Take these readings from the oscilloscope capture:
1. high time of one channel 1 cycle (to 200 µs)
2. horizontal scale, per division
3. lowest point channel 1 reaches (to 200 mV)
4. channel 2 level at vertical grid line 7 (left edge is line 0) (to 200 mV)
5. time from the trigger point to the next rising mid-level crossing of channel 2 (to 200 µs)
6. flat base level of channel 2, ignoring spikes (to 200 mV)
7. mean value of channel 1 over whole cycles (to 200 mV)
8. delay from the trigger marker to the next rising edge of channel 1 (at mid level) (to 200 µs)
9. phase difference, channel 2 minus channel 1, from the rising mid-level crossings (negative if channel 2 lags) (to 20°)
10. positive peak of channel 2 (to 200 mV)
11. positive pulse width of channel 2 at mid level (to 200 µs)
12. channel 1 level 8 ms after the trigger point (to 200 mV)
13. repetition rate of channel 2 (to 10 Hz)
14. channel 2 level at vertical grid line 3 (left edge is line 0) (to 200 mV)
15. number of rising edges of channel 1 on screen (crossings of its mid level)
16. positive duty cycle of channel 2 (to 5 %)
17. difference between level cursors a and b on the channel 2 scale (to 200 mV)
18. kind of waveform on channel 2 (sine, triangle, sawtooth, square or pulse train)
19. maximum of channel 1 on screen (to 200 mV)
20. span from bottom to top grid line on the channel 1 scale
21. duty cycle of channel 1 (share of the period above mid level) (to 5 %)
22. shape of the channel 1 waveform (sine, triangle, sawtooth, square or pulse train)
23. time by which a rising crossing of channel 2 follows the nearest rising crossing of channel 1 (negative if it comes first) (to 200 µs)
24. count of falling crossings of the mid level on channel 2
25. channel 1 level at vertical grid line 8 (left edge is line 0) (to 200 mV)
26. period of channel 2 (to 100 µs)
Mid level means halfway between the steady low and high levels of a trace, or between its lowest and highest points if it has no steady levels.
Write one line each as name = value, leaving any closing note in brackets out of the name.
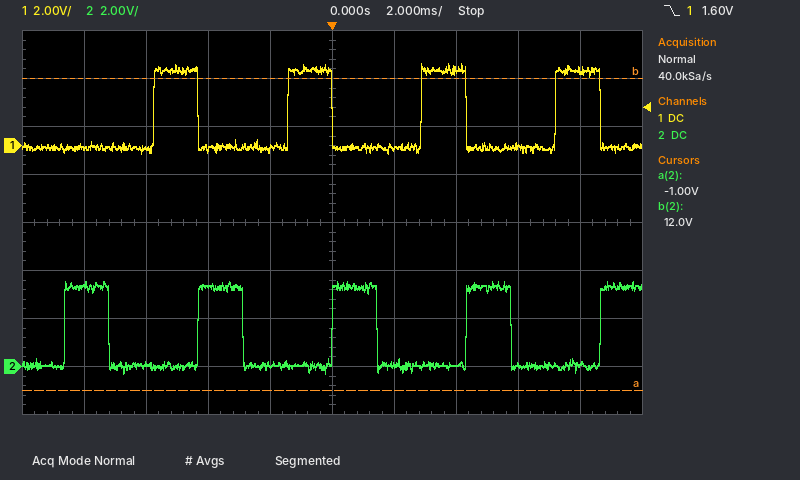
high time of one channel 1 cycle = 1.4 ms
horizontal scale, per division = 2 ms
lowest point channel 1 reaches = -400 mV
channel 2 level at vertical grid line 7 (left edge is line 0) = 0.0 V
time from the trigger point to the next rising mid-level crossing of channel 2 = 4.4 ms
flat base level of channel 2, ignoring spikes = 0.0 V
mean value of channel 1 over whole cycles = 1.0 V
delay from the trigger marker to the next rising edge of channel 1 (at mid level) = 2.8 ms
phase difference, channel 2 minus channel 1, from the rising mid-level crossings (negative if channel 2 lags) = -120°
positive peak of channel 2 = 3.6 V
positive pulse width of channel 2 at mid level = 1.4 ms
channel 1 level 8 ms after the trigger point = 3.2 V
repetition rate of channel 2 = 230 Hz
channel 2 level at vertical grid line 3 (left edge is line 0) = 3.4 V
number of rising edges of channel 1 on screen = 4
positive duty cycle of channel 2 = 35 %
difference between level cursors a and b on the channel 2 scale = 13.0 V
kind of waveform on channel 2 = pulse train
maximum of channel 1 on screen = 3.4 V
span from bottom to top grid line on the channel 1 scale = 16 V
duty cycle of channel 1 (share of the period above mid level) = 35 %
shape of the channel 1 waveform = pulse train
time by which a rising crossing of channel 2 follows the nearest rising crossing of channel 1 (negative if it comes first) = +1.4 ms
count of falling crossings of the mid level on channel 2 = 4
channel 1 level at vertical grid line 8 (left edge is line 0) = 0.0 V
period of channel 2 = 4.3 ms
